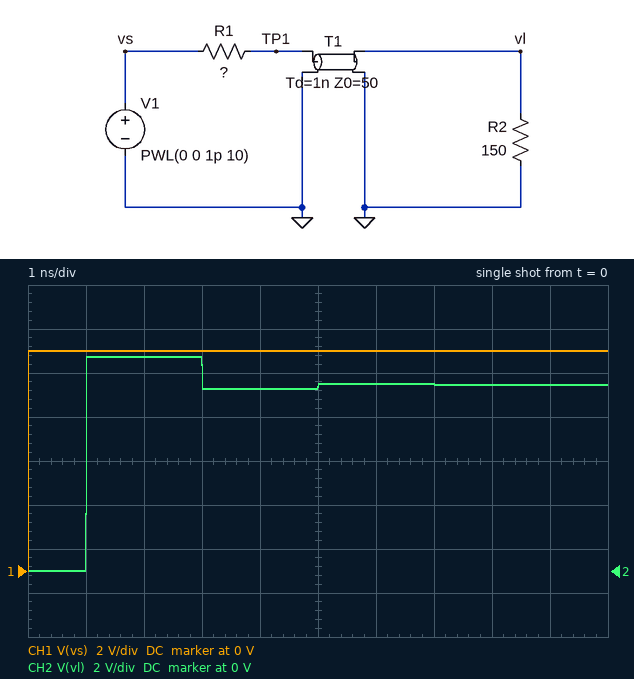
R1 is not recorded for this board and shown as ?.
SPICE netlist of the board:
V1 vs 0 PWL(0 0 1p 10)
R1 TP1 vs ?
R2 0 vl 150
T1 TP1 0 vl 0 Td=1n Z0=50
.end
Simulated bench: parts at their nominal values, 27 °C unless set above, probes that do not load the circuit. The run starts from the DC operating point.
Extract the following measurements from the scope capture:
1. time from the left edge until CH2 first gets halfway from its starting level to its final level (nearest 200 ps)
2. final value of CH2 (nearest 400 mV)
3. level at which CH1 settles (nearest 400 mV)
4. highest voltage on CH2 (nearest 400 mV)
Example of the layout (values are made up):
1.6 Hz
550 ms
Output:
1.0 ns
8.4 V
10.0 V
9.6 V
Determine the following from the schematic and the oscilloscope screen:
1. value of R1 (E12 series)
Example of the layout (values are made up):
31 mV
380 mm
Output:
27 Ω
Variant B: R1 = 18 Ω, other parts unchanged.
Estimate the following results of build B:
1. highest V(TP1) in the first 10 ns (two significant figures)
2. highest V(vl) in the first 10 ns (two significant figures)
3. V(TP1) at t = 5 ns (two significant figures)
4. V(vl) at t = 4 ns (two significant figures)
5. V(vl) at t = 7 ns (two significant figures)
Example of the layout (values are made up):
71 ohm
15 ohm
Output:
9.3 V
11 V
8.8 V
8.4 V
9.0 V
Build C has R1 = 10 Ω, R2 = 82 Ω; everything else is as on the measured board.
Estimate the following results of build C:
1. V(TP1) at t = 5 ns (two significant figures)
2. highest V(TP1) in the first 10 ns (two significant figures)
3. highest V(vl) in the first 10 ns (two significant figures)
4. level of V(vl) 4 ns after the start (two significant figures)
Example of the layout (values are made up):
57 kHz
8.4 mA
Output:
8.9 V
9.0 V
10 V
8.7 V
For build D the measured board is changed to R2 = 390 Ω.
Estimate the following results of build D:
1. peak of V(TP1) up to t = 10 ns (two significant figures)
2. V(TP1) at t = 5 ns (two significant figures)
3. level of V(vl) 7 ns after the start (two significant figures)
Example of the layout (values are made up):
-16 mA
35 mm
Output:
10 V
9.2 V
9.4 V
